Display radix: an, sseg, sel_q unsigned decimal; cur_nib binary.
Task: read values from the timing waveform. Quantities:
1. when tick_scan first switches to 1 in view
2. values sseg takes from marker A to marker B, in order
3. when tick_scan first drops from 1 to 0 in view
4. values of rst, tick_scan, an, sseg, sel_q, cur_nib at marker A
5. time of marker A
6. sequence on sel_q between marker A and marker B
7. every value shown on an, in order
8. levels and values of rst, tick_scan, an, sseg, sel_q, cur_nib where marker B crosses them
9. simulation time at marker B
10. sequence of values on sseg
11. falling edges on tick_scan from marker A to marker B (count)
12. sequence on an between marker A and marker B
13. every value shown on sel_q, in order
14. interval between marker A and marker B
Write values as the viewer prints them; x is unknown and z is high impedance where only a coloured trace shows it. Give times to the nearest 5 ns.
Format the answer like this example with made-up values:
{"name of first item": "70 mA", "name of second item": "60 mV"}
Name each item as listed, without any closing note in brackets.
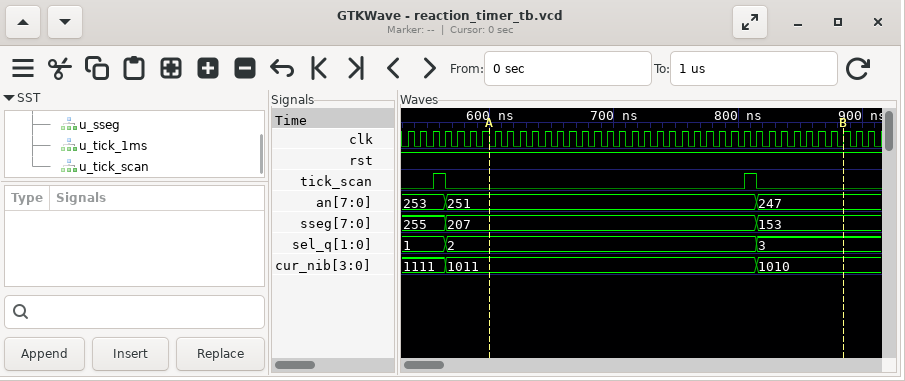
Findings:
{"when tick_scan first switches to 1 in view": "555 ns", "values sseg takes from marker A to marker B, in order": "207, 153", "when tick_scan first drops from 1 to 0 in view": "565 ns", "values of rst, tick_scan, an, sseg, sel_q, cur_nib at marker A": "rst=1, tick_scan=0, an=251, sseg=207, sel_q=2, cur_nib=1011", "time of marker A": "600 ns", "sequence on sel_q between marker A and marker B": "2, 3", "every value shown on an, in order": "253, 251, 247", "levels and values of rst, tick_scan, an, sseg, sel_q, cur_nib where marker B crosses them": "rst=1, tick_scan=0, an=247, sseg=153, sel_q=3, cur_nib=1010", "simulation time at marker B": "885 ns", "sequence of values on sseg": "255, 207, 153", "falling edges on tick_scan from marker A to marker B": "1", "sequence on an between marker A and marker B": "251, 247", "every value shown on sel_q, in order": "1, 2, 3", "interval between marker A and marker B": "285 ns"}
